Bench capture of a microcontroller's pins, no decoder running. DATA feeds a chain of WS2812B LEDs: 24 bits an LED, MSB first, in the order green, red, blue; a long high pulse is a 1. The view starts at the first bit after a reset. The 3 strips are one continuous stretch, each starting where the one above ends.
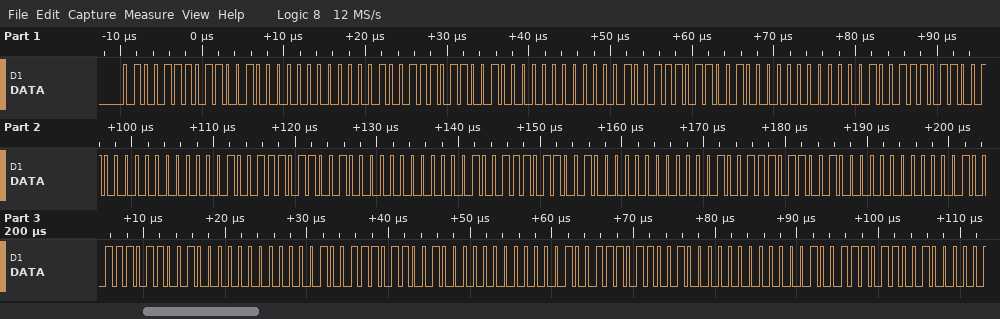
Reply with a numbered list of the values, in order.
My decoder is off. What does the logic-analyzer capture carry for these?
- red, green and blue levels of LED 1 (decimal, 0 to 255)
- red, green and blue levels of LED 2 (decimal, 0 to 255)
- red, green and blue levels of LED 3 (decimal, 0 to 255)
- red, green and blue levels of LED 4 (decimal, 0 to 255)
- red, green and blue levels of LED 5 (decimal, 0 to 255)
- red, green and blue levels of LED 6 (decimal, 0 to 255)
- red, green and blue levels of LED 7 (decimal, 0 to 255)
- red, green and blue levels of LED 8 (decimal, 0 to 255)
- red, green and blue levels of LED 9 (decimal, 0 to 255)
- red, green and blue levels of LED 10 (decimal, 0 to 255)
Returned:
1. 200, 78, 0
2. 200, 78, 0
3. 200, 78, 0
4. 200, 78, 0
5. 200, 78, 0
6. 200, 78, 0
7. 200, 78, 0
8. 200, 78, 0
9. 200, 78, 0
10. 200, 78, 0
